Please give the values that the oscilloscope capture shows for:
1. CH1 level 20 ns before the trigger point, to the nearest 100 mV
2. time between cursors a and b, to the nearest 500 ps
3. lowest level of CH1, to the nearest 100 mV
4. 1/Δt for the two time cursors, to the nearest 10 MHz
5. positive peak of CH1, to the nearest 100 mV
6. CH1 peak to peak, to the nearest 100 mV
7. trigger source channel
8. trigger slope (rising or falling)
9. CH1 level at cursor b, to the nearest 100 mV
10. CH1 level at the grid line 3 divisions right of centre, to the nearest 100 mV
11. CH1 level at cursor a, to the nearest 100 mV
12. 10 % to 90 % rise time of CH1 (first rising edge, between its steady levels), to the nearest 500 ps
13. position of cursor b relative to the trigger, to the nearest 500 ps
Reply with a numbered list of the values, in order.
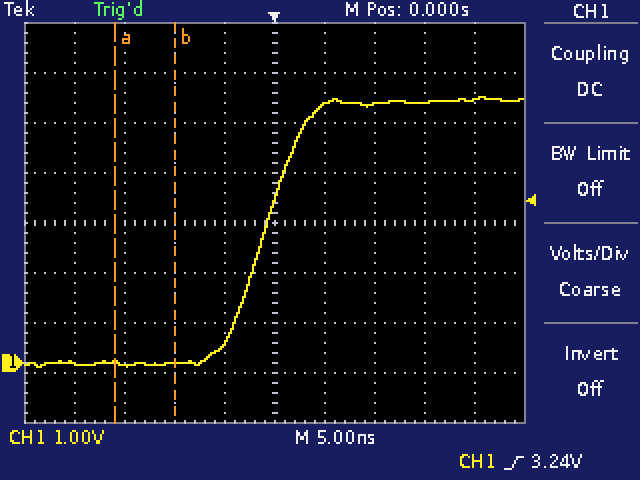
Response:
1. 0.0 V
2. 6.0 ns
3. -100 mV
4. 170 MHz
5. 5.3 V
6. 5.4 V
7. CH1
8. rising
9. 0.0 V
10. 5.2 V
11. 0.0 V
12. 7.5 ns
13. -10.0 ns
